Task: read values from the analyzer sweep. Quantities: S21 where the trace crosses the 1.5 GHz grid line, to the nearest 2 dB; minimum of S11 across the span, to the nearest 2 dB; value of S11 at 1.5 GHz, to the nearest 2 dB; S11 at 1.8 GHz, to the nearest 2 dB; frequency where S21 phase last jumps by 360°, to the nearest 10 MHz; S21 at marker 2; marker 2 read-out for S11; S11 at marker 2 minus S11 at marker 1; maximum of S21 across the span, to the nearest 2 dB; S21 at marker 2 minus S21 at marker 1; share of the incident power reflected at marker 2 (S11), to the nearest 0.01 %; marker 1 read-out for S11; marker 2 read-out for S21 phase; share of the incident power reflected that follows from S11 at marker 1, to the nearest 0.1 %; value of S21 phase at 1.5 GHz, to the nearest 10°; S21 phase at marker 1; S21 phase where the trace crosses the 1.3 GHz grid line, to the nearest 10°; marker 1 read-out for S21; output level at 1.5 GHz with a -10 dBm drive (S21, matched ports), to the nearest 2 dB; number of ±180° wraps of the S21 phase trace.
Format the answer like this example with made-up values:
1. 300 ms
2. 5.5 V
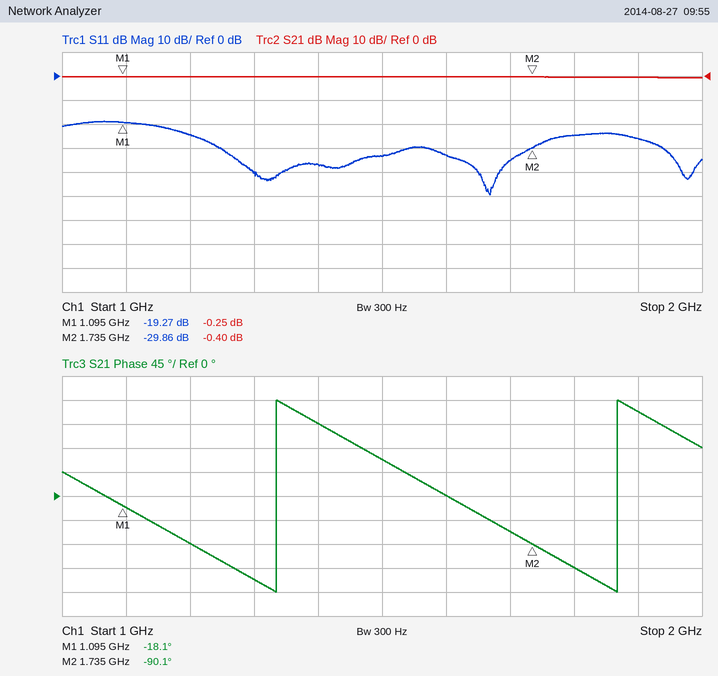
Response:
1. 0 dB
2. -50 dB
3. -34 dB
4. -24 dB
5. 1.87 GHz
6. -0.40 dB
7. -29.86 dB
8. -10.59 dB
9. 0 dB
10. -0.15 dB
11. 0.10 %
12. -19.27 dB
13. -90.1°
14. 1.2 %
15. 70°
16. -18.1°
17. -160°
18. -0.25 dB
19. -10 dBm
20. 2
